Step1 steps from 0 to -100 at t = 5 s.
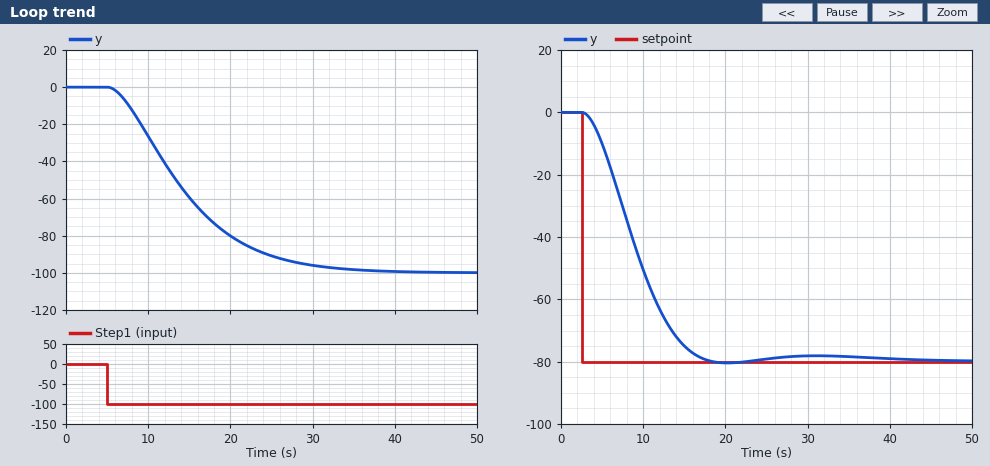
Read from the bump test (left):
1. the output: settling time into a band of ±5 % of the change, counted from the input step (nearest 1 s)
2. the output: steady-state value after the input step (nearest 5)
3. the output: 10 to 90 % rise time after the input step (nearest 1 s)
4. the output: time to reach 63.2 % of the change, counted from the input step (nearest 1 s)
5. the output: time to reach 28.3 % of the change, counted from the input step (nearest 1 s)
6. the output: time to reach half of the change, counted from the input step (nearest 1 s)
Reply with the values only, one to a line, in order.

24 s
-100
17 s
11 s
5 s
8 s
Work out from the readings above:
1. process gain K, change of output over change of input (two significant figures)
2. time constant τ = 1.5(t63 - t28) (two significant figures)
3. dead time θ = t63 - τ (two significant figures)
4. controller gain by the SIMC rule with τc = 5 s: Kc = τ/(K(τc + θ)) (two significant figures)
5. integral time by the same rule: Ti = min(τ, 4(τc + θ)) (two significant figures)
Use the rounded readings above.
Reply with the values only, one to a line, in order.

1.0
9.0 s
2.0 s
1.3
9.0 s
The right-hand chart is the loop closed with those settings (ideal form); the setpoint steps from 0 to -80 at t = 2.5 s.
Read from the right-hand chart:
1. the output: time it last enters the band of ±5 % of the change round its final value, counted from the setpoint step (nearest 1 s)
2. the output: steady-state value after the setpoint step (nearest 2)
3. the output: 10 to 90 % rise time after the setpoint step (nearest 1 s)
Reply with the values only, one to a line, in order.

13 s
-80
9 s
